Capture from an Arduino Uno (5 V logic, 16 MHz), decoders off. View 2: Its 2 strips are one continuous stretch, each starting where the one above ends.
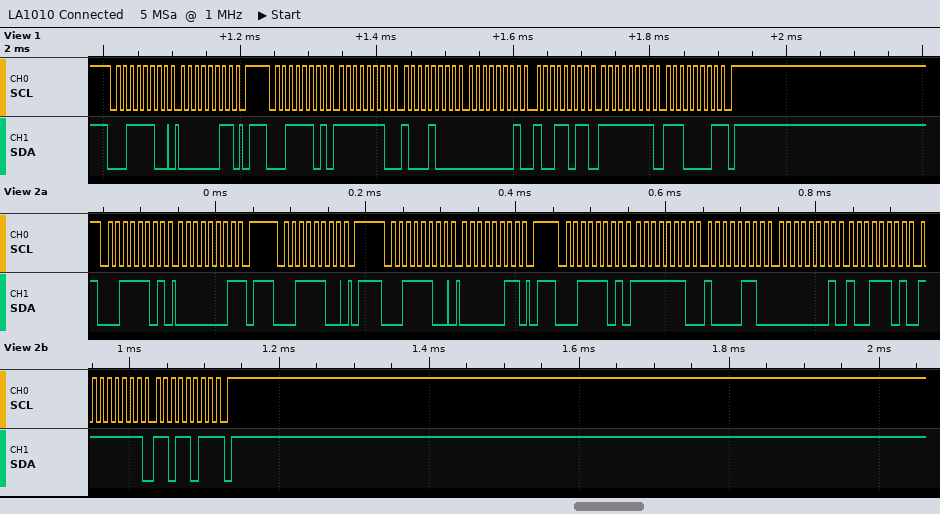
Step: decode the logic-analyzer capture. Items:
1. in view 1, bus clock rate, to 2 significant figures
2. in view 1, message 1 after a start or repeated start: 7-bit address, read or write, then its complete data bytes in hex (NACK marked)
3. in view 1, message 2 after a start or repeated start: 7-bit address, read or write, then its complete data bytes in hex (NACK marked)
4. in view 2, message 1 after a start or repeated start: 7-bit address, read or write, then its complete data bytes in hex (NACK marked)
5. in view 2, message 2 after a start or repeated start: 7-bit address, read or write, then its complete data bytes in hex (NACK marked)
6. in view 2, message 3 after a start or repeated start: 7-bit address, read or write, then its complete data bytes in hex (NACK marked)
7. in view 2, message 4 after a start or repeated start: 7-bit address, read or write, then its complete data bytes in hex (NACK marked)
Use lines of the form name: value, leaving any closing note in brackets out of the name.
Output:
in view 1, bus clock rate, to 2 significant figures: 100 kHz
in view 1, message 1 after a start or repeated start: 7-bit address, read or write, then its complete data bytes in hex: 0x1E write: 03
in view 1, message 2 after a start or repeated start: 7-bit address, read or write, then its complete data bytes in hex: 0x1E read: FE 88 01 9B FF E1 NACK
in view 2, message 1 after a start or repeated start: 7-bit address, read or write, then its complete data bytes in hex: 0x1E read: 01 NACK
in view 2, message 2 after a start or repeated start: 7-bit address, read or write, then its complete data bytes in hex: 0x1E write
in view 2, message 3 after a start or repeated start: 7-bit address, read or write, then its complete data bytes in hex: 0x1E write: 03
in view 2, message 4 after a start or repeated start: 7-bit address, read or write, then its complete data bytes in hex: 0x1E read: FE 86 01 9D FF DB NACK
